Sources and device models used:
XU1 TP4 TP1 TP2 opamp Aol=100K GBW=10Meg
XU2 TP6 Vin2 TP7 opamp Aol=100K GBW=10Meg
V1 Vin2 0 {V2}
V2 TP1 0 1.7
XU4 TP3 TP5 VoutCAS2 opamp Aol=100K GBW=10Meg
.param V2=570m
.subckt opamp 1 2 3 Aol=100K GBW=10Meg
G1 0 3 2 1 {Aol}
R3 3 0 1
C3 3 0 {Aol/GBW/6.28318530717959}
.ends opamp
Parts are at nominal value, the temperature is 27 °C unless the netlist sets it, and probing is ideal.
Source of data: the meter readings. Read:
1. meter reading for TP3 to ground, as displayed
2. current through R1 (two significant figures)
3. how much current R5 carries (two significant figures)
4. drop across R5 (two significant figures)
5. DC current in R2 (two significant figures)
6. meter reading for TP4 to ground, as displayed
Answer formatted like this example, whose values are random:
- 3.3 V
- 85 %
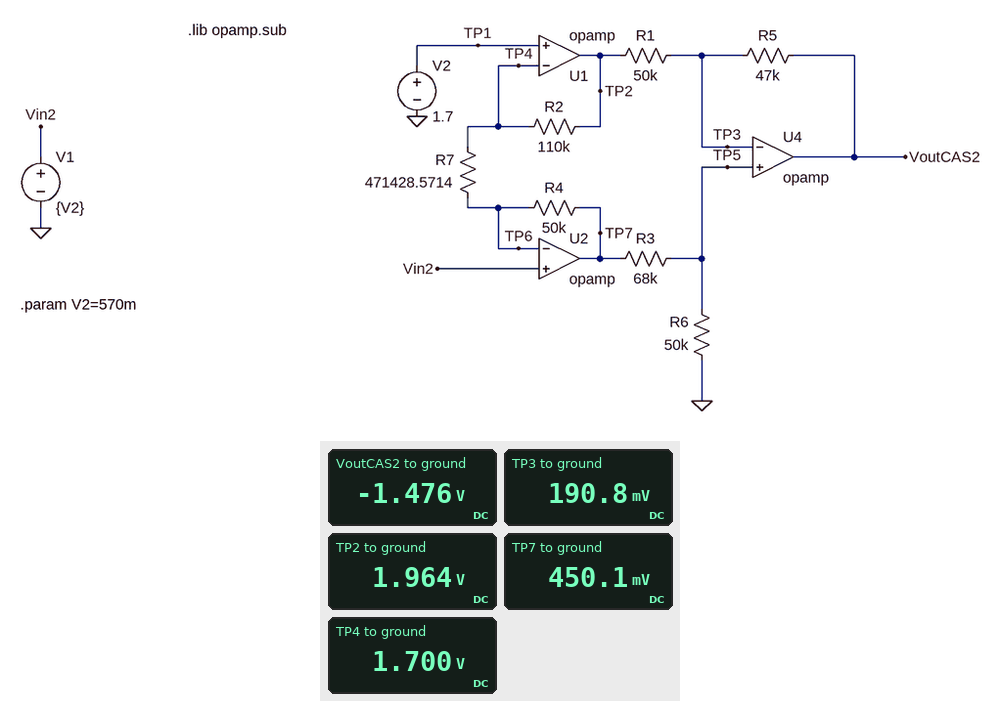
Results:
- 190.8 mV
- 35 µA
- 35 µA
- 1.7 V
- 2.4 µA
- 1.700 V
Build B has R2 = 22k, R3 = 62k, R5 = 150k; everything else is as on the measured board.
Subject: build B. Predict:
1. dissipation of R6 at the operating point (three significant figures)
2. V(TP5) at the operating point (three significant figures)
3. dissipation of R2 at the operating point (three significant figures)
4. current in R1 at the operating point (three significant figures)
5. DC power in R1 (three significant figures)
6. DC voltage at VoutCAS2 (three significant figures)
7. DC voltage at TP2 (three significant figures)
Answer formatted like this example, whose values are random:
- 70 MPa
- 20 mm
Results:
- 808 nW
- 201 mV
- 126 nW
- 31.0 µA
- 48.2 µW
- -4.45 V
- 1.75 V
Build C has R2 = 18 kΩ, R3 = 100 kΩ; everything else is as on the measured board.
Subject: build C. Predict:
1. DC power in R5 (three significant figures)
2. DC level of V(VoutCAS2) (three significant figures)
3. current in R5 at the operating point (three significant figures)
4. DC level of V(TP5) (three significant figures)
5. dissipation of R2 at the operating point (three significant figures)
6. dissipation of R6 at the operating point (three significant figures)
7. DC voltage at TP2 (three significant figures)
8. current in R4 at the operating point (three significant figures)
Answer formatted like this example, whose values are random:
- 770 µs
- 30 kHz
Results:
- 47.7 µW
- -1.35 V
- 31.9 µA
- 150 mV
- 103 nW
- 450 nW
- 1.74 V
- 2.40 µA
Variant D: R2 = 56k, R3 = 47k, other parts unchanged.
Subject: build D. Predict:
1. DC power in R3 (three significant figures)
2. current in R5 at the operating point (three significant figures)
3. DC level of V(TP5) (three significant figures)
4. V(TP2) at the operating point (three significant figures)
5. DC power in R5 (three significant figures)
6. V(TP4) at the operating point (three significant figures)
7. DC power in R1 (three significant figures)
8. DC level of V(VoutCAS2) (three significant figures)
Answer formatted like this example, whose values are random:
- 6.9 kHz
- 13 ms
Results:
- 1.01 µW
- 32.0 µA
- 232 mV
- 1.83 V
- 48.3 µW
- 1.70 V
- 51.3 µW
- -1.27 V
